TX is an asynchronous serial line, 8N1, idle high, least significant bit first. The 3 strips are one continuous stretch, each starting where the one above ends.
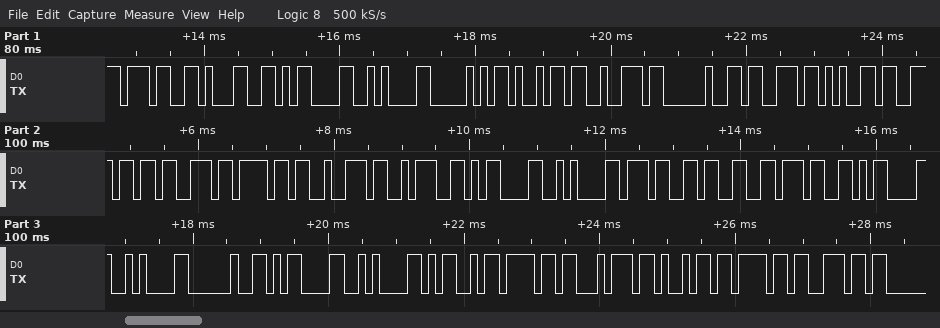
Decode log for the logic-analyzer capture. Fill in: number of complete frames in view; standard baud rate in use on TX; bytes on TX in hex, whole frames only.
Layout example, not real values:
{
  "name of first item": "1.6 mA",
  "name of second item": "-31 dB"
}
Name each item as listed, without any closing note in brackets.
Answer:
{
  "number of complete frames in view": "31",
  "standard baud rate in use on TX": "9600 baud",
  "bytes on TX in hex, whole frames only": "37 31 0D 0A 50 69 72 20 73 65 6E 73 6F 72 3A 0D 0A 37 33 37 0D 0A 20 0D 0A 4D 6F 74 69 6F 6E"
}
